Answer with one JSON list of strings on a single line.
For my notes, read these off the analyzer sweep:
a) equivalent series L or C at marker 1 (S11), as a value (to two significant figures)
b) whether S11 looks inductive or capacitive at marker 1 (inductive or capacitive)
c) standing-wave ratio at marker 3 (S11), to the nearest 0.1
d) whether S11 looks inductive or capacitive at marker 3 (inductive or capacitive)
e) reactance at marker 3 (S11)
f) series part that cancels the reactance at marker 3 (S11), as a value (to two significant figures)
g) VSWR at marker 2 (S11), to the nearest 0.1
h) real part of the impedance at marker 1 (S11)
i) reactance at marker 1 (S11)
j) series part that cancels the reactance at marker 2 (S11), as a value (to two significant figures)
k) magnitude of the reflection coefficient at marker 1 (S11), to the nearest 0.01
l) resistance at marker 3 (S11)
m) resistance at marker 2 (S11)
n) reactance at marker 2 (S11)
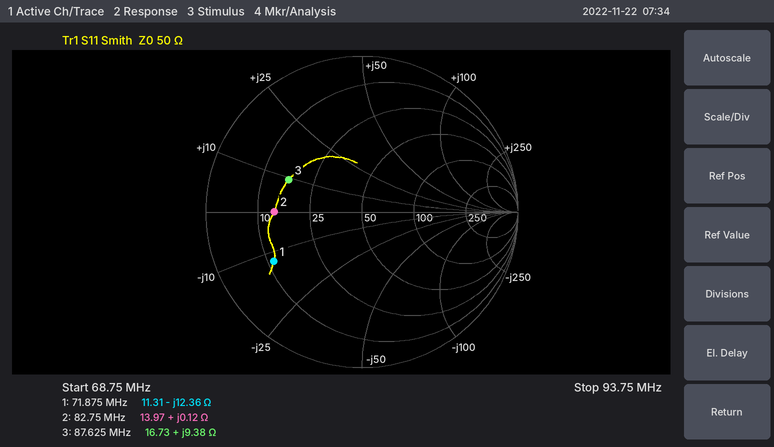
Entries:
["180 pF", "capacitive", "3.1", "inductive", "+9.38 Ω", "190 pF", "3.6", "11.31 Ω", "-12.36 Ω", "16 nF", "0.65", "16.73 Ω", "13.97 Ω", "+0.12 Ω"]
